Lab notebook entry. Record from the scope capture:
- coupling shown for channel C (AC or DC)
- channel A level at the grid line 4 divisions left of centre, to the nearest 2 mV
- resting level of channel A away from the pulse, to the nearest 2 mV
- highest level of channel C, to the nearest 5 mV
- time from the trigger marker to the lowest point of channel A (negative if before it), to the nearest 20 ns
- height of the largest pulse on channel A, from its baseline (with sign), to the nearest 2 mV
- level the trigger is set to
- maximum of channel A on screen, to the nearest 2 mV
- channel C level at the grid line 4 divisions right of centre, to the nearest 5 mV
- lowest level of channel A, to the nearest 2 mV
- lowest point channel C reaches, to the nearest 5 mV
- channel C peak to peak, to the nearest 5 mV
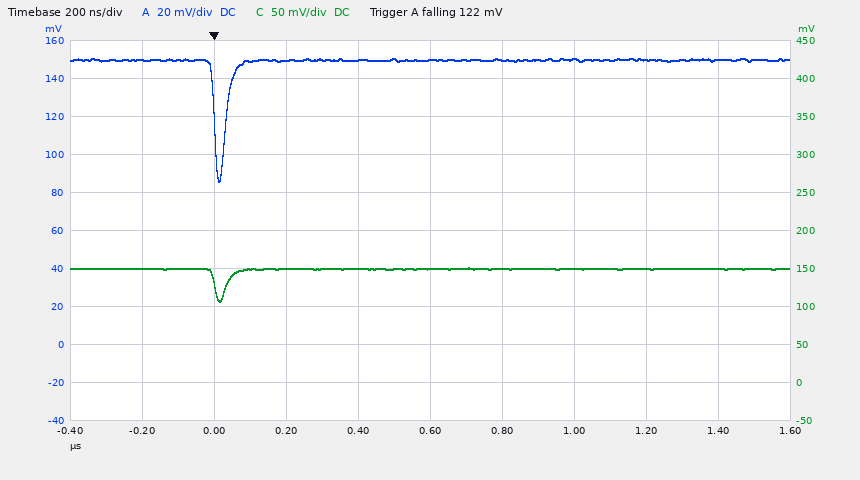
DC
150 mV
150 mV
150 mV
+20 ns
-64 mV
122 mV
150 mV
150 mV
86 mV
105 mV
45 mV
